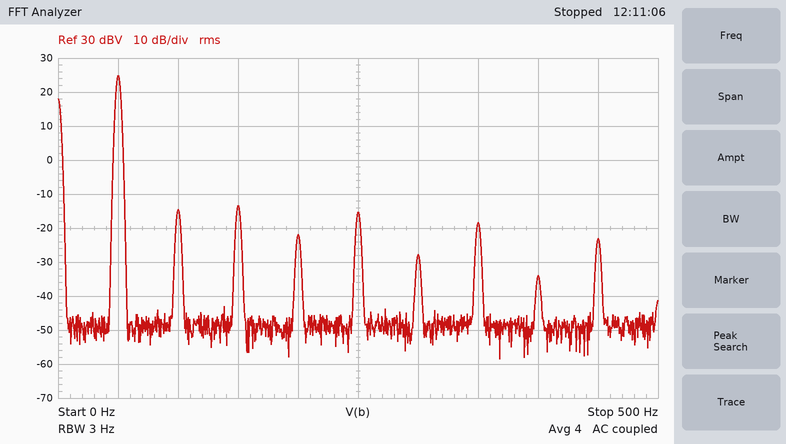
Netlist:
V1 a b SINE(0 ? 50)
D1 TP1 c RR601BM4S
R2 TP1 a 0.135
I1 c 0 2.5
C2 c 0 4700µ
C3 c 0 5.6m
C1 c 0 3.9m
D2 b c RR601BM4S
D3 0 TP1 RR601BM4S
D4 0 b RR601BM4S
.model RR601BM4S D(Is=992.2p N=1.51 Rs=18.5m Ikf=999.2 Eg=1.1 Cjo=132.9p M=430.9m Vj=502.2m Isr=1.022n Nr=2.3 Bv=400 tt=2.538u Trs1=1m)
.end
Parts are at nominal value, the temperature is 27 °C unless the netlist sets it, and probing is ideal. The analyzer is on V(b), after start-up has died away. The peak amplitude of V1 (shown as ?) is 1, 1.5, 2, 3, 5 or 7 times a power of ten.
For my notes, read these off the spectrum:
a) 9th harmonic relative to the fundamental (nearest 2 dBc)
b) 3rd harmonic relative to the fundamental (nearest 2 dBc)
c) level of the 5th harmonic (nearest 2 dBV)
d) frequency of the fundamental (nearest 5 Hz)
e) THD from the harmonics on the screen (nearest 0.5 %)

-48 dBc
-38 dBc
-16 dBV
50 Hz
2.0 %
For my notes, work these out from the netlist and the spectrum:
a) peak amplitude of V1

50 V
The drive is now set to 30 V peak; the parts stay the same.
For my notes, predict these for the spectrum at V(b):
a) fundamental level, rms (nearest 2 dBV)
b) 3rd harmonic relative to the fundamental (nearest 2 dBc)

20 dBV
-34 dBc
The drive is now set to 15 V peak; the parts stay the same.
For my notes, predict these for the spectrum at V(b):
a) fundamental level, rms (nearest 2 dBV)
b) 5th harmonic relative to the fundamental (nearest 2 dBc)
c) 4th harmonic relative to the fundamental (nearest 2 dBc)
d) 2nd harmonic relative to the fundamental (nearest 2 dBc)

14 dBV
-34 dBc
-38 dBc
-30 dBc
